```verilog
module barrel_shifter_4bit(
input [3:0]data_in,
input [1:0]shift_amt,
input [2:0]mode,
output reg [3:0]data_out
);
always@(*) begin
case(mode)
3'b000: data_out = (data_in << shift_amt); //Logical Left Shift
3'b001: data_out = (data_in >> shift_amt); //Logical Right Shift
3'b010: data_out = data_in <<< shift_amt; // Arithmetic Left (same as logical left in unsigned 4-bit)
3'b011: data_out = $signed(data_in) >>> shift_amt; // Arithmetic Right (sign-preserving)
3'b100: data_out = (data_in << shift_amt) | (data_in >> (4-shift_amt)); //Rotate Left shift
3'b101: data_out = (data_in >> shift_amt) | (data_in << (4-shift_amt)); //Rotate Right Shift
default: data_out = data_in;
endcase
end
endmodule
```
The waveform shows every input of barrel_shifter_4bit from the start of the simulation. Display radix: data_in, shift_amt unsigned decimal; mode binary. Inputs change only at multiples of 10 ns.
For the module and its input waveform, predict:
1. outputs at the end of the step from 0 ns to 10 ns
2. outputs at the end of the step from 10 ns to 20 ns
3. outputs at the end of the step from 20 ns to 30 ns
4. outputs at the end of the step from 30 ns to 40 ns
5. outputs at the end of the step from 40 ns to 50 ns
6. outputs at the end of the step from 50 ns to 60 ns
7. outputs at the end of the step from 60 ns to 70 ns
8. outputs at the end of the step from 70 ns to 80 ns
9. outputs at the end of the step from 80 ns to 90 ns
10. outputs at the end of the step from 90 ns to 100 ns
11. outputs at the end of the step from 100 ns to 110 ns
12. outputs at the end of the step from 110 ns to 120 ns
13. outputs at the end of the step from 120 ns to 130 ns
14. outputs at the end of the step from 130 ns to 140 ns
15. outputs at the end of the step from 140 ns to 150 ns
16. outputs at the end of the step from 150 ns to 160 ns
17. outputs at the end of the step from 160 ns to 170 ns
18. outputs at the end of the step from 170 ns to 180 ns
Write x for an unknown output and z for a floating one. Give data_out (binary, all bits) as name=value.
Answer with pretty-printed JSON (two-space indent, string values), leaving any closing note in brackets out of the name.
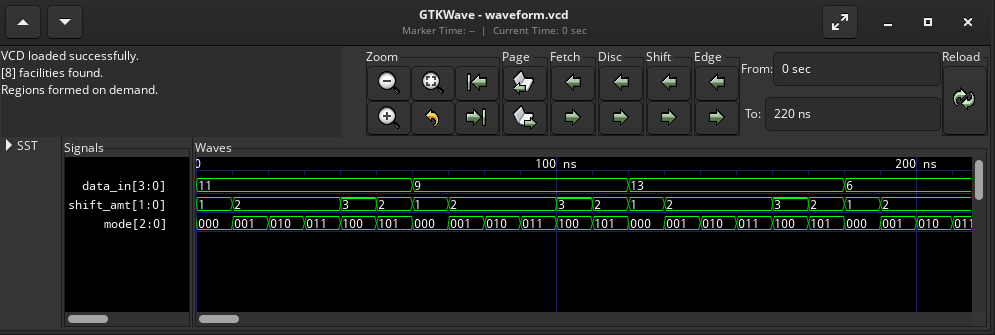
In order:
{
  "outputs at the end of the step from 0 ns to 10 ns": "data_out=0110",
  "outputs at the end of the step from 10 ns to 20 ns": "data_out=0010",
  "outputs at the end of the step from 20 ns to 30 ns": "data_out=1100",
  "outputs at the end of the step from 30 ns to 40 ns": "data_out=1110",
  "outputs at the end of the step from 40 ns to 50 ns": "data_out=1101",
  "outputs at the end of the step from 50 ns to 60 ns": "data_out=1110",
  "outputs at the end of the step from 60 ns to 70 ns": "data_out=0010",
  "outputs at the end of the step from 70 ns to 80 ns": "data_out=0010",
  "outputs at the end of the step from 80 ns to 90 ns": "data_out=0100",
  "outputs at the end of the step from 90 ns to 100 ns": "data_out=1110",
  "outputs at the end of the step from 100 ns to 110 ns": "data_out=1100",
  "outputs at the end of the step from 110 ns to 120 ns": "data_out=0110",
  "outputs at the end of the step from 120 ns to 130 ns": "data_out=1010",
  "outputs at the end of the step from 130 ns to 140 ns": "data_out=0011",
  "outputs at the end of the step from 140 ns to 150 ns": "data_out=0100",
  "outputs at the end of the step from 150 ns to 160 ns": "data_out=1111",
  "outputs at the end of the step from 160 ns to 170 ns": "data_out=1110",
  "outputs at the end of the step from 170 ns to 180 ns": "data_out=0111"
}
